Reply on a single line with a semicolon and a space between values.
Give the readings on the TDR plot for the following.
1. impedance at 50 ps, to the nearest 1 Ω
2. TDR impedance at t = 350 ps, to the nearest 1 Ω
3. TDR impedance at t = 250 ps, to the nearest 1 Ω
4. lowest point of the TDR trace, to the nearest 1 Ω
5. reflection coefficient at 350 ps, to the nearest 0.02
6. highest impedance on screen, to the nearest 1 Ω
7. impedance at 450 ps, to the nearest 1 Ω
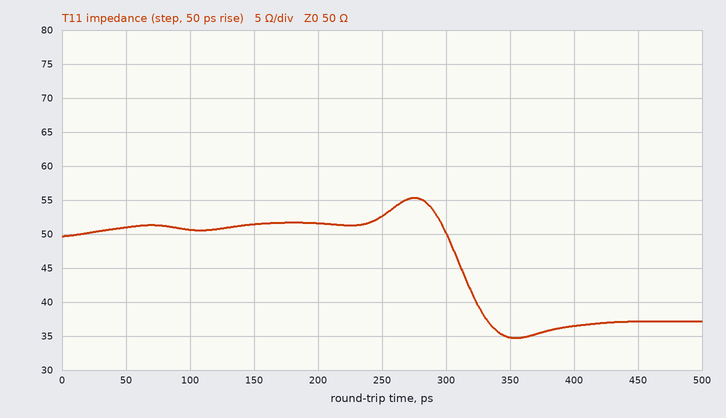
51 Ω; 35 Ω; 53 Ω; 35 Ω; -0.18; 55 Ω; 37 Ω
